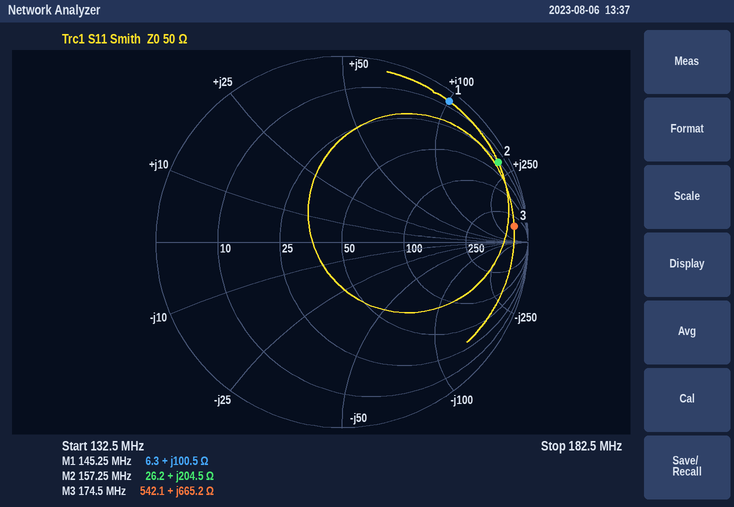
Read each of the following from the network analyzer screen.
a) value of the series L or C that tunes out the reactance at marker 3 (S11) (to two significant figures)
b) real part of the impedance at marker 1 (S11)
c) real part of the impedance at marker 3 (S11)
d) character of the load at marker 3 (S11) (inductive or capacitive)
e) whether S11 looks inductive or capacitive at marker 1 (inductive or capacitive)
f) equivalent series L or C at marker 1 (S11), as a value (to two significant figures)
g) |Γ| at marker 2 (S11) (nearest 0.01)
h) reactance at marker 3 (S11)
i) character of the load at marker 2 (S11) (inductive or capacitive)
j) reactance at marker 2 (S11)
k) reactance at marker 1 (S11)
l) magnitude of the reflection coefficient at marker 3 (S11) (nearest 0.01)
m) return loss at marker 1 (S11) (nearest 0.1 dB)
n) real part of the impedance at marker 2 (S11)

1.4 pF
6.3 Ω
542.1 Ω
inductive
inductive
110 nH
0.94
+665.2 Ω
inductive
+204.5 Ω
+100.5 Ω
0.93
0.4 dB
26.2 Ω
